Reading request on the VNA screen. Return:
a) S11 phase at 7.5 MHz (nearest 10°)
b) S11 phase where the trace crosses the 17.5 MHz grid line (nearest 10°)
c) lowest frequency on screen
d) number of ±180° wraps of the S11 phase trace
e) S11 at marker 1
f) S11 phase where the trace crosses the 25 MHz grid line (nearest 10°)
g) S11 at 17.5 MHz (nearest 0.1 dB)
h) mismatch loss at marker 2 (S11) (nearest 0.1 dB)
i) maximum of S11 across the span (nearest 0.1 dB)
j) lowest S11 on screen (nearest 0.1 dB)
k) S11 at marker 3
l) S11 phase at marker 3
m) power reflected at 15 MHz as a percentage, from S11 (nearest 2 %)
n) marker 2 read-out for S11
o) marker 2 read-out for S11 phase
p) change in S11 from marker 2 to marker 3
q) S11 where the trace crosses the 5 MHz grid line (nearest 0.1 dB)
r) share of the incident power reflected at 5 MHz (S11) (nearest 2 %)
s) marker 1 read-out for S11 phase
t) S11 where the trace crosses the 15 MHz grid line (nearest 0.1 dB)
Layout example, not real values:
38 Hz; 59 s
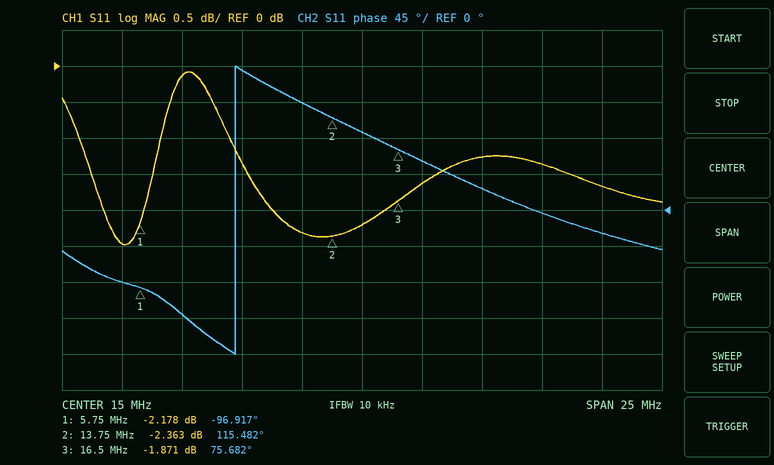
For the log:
-130°; 60°; 2.5 MHz; 1; -2.178 dB; -30°; -1.6 dB; 3.8 dB; -0.1 dB; -2.5 dB; -1.871 dB; 75.682°; 60 %; -2.363 dB; 115.482°; 0.492 dB; -2.5 dB; 56 %; -96.917°; -2.2 dB
